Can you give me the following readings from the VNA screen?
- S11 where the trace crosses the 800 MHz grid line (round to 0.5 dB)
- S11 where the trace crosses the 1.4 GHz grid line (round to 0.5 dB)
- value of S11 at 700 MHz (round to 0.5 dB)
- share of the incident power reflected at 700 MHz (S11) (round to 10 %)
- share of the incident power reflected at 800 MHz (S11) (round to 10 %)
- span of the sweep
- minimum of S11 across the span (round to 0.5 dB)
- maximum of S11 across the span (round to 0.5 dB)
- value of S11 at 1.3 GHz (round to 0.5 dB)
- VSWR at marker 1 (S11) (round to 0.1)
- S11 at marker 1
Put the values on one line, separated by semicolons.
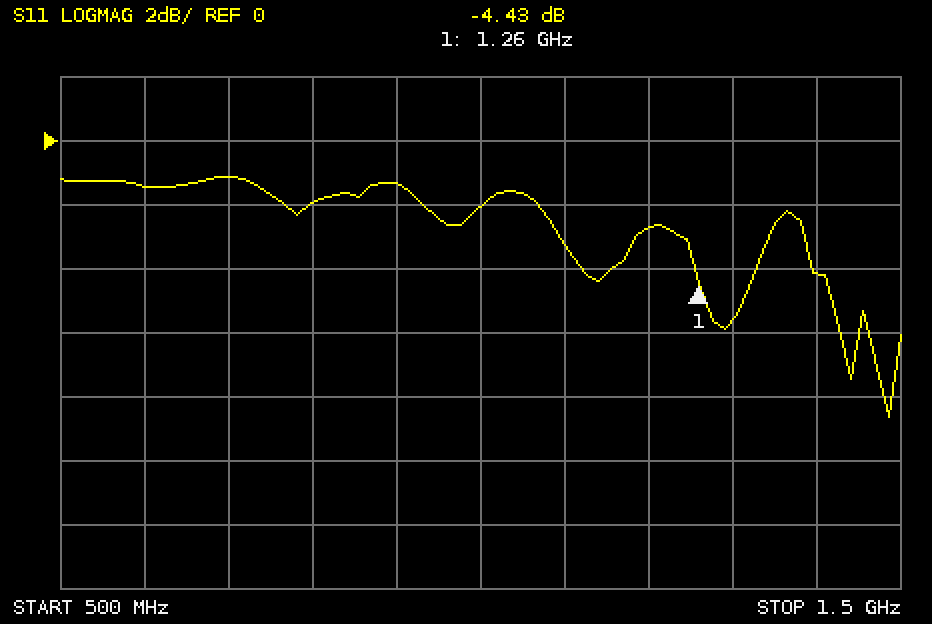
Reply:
-2.0 dB; -4.0 dB; -1.0 dB; 80 %; 60 %; 1 GHz; -8.5 dB; -1.0 dB; -5.5 dB; 4.0; -4.43 dB
